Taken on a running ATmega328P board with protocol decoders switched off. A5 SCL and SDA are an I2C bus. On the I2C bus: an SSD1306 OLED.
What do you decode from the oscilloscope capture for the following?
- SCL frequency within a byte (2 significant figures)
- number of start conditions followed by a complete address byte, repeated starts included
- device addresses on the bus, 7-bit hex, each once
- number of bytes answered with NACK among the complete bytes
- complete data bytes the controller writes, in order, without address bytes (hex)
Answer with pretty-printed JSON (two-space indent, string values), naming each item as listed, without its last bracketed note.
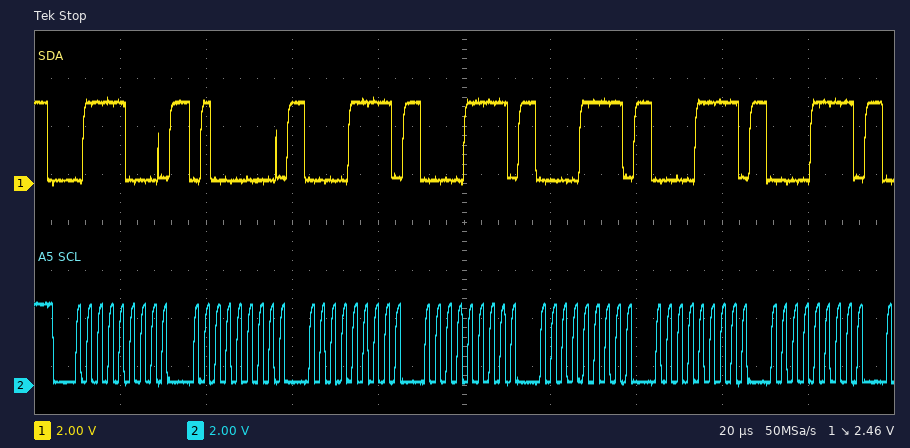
{
  "SCL frequency within a byte": "400 kHz",
  "number of start conditions followed by a complete address byte, repeated starts included": "1",
  "device addresses on the bus, 7-bit hex, each once": "0x3C",
  "number of bytes answered with NACK among the complete bytes": "0",
  "complete data bytes the controller writes, in order, without address bytes": "40 0F 0F 0F 0F 0F"
}
